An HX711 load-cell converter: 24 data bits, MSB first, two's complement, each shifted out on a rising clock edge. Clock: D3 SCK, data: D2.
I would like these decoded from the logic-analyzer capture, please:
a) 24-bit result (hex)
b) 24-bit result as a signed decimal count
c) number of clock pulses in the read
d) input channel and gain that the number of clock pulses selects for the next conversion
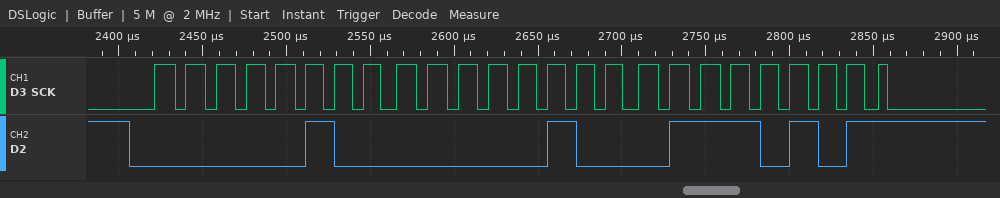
0x040475
263285
25
channel A, gain 128
